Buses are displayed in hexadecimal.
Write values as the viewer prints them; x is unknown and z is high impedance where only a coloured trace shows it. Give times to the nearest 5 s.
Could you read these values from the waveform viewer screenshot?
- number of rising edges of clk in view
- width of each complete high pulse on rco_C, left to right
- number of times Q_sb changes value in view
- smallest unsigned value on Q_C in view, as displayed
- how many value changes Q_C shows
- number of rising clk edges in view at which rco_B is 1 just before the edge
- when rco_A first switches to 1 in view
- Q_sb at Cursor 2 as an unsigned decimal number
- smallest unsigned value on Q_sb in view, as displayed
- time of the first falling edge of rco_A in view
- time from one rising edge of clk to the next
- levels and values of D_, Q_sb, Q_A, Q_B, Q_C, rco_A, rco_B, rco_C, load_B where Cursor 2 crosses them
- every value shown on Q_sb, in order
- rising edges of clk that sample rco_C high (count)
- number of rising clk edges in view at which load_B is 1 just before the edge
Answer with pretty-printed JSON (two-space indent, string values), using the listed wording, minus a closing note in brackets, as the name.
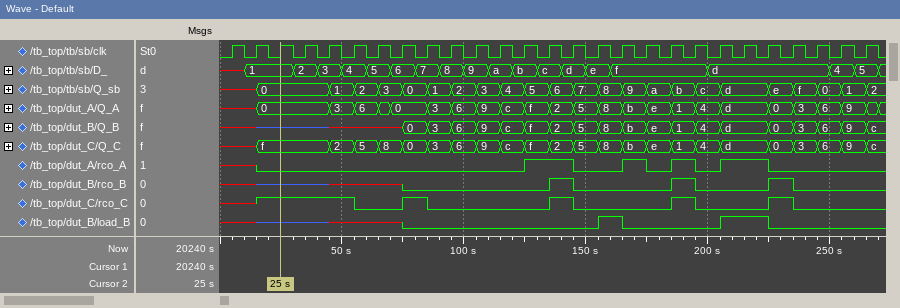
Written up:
{
  "number of rising edges of clk in view": "27",
  "width of each complete high pulse on rco_C, left to right": "10 s, 10 s, 10 s, 10 s",
  "number of times Q_sb changes value in view": "23",
  "smallest unsigned value on Q_C in view, as displayed": "0",
  "how many value changes Q_C shows": "23",
  "number of rising clk edges in view at which rco_B is 1 just before the edge": "3",
  "when rco_A first switches to 1 in view": "125 s",
  "Q_sb at Cursor 2 as an unsigned decimal number": "0",
  "smallest unsigned value on Q_sb in view, as displayed": "0",
  "time of the first falling edge of rco_A in view": "145 s",
  "time from one rising edge of clk to the next": "10 s",
  "levels and values of D_, Q_sb, Q_A, Q_B, Q_C, rco_A, rco_B, rco_C, load_B where Cursor 2 crosses them": "D_=1, Q_sb=0, Q_A=0, Q_B=z, Q_C=f, rco_A=0, rco_B=z, rco_C=1, load_B=z",
  "every value shown on Q_sb, in order": "x, 0, 1, 2, 3, 0, 1, 2, 3, 4, 5, 6, 7, 8, 9, a, b, c, d, e, f, 0, 1, 2",
  "rising edges of clk that sample rco_C high": "8",
  "number of rising clk edges in view at which load_B is 1 just before the edge": "3"
}
